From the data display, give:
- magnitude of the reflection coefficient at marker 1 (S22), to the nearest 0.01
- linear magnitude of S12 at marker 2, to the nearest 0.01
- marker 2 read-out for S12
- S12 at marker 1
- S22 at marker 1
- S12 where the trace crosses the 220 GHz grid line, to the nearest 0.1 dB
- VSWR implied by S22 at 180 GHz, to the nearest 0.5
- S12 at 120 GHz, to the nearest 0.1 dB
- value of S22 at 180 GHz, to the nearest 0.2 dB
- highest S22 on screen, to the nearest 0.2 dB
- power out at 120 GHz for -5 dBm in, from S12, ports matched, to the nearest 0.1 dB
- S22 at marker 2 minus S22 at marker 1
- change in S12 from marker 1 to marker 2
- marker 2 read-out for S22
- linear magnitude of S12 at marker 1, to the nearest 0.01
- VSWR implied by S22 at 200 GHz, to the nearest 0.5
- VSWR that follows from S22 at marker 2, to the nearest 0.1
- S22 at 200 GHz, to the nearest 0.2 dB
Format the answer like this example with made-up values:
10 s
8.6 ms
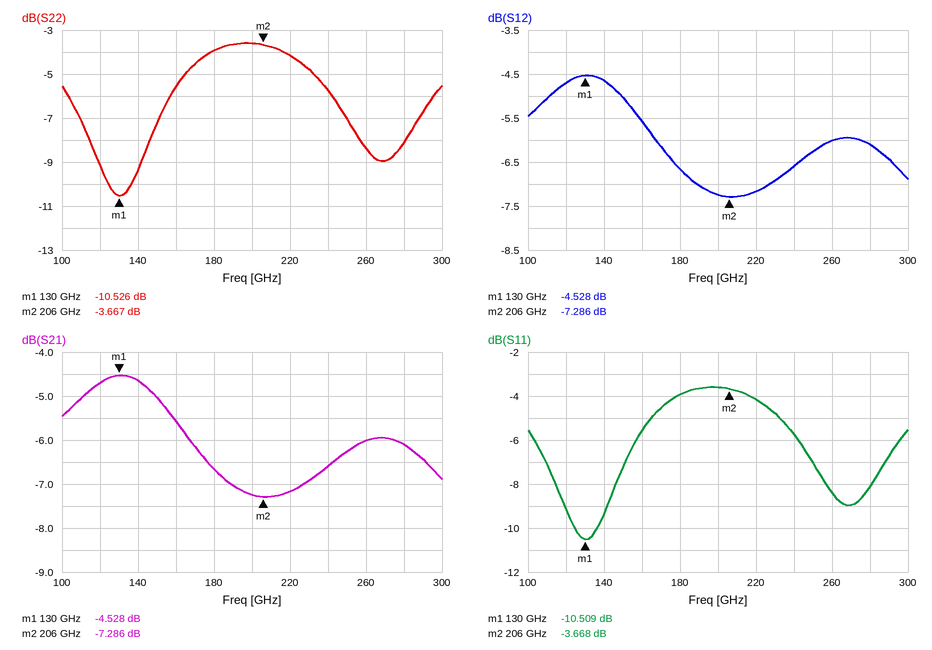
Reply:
0.30
0.43
-7.286 dB
-4.528 dB
-10.526 dB
-7.2 dB
4.5
-4.7 dB
-4.0 dB
-3.6 dB
-9.7 dBm
6.859 dB
-2.758 dB
-3.667 dB
0.59
5.0
4.8
-3.6 dB
